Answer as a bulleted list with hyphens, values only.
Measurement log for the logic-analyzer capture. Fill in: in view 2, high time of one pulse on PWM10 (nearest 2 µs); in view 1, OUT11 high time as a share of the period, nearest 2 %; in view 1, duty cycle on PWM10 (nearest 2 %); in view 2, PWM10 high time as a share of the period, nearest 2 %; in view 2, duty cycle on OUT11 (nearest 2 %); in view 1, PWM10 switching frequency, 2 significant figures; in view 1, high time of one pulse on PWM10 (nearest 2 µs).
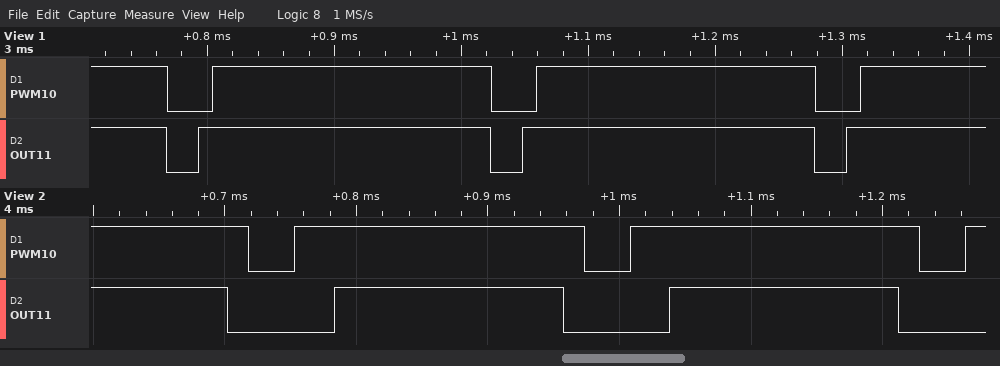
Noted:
- 220 µs
- 90 %
- 86 %
- 86 %
- 68 %
- 3.9 kHz
- 220 µs
